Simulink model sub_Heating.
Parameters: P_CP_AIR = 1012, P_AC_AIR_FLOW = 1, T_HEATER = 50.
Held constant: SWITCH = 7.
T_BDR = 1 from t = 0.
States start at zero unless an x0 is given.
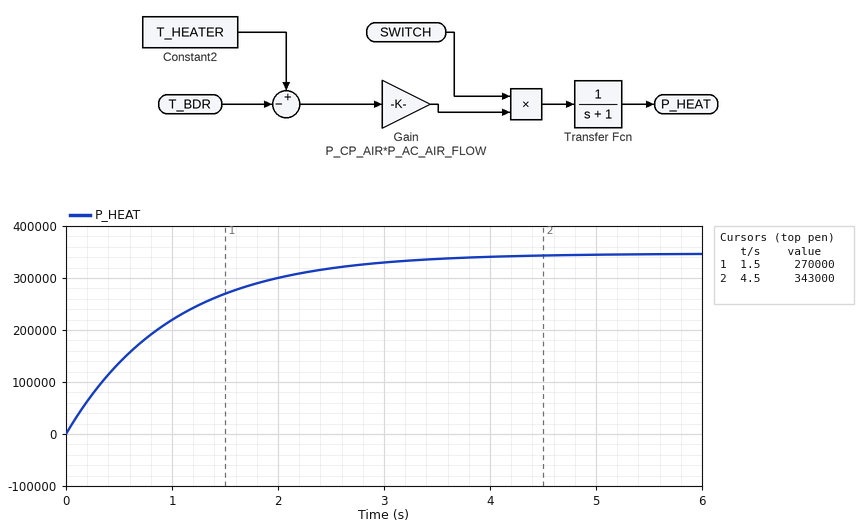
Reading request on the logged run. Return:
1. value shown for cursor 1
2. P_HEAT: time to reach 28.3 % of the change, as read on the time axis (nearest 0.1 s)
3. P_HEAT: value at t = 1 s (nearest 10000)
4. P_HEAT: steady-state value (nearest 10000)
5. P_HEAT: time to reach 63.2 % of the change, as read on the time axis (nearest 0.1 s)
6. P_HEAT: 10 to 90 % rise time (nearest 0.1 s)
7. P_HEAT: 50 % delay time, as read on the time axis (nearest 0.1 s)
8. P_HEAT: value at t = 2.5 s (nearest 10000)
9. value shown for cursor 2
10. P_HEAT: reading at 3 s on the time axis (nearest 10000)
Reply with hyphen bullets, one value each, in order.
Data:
- 270000
- 0.3 s
- 220000
- 350000
- 1.0 s
- 2.2 s
- 0.7 s
- 320000
- 343000
- 330000
